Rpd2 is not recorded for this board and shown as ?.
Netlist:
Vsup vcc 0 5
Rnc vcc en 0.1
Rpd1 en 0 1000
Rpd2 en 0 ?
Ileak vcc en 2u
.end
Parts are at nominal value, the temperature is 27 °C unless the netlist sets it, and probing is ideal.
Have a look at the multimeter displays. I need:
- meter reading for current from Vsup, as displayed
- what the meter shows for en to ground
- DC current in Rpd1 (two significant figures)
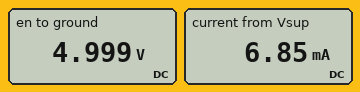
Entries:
6.85 mA
4.999 V
5.0 mA
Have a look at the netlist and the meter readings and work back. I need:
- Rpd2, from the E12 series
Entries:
2.7 kΩ
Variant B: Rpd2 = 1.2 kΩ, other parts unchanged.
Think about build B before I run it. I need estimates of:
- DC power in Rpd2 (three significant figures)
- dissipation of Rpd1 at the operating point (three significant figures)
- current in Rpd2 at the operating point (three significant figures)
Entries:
20.8 mW
25.0 mW
4.17 mA
